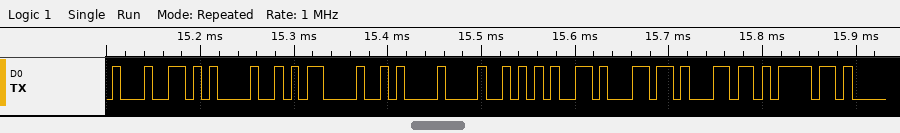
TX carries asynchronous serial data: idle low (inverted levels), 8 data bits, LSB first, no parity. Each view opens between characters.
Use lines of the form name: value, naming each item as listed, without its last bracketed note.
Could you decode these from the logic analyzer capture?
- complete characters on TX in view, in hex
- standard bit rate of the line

complete characters on TX in view, in hex: 37, BD, E5, EB, 6F, 35, 27, 27, 21
standard bit rate of the line: 115200 baud
